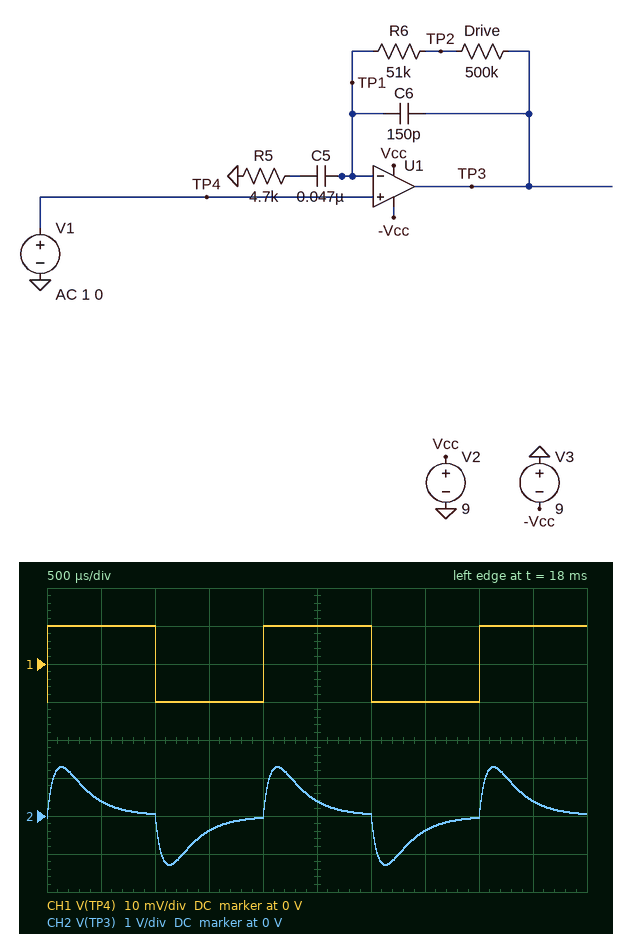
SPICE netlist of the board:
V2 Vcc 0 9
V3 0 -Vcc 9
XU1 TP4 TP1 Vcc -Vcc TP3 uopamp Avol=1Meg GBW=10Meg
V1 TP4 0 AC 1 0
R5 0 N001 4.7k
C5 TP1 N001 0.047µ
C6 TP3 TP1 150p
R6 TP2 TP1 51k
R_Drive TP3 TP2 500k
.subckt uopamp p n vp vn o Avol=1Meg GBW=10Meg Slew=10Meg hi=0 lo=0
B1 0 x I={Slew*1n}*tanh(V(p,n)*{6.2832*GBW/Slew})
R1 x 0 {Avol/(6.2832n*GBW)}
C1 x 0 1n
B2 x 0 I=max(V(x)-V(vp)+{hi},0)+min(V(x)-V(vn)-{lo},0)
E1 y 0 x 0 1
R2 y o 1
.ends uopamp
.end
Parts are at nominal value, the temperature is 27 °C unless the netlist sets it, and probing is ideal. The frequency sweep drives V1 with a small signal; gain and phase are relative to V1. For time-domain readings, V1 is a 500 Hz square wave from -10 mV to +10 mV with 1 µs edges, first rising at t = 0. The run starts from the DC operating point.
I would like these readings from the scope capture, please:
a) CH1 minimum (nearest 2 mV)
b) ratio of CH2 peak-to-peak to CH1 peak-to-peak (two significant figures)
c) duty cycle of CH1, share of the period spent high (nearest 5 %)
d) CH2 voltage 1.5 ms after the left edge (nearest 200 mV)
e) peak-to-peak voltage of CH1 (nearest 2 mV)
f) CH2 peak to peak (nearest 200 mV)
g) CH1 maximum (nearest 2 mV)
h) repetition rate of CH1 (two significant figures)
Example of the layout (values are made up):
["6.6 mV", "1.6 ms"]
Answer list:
["-10 mV", "130", "50 %", "-400 mV", "20 mV", "2.6 V", "10 mV", "500 Hz"]
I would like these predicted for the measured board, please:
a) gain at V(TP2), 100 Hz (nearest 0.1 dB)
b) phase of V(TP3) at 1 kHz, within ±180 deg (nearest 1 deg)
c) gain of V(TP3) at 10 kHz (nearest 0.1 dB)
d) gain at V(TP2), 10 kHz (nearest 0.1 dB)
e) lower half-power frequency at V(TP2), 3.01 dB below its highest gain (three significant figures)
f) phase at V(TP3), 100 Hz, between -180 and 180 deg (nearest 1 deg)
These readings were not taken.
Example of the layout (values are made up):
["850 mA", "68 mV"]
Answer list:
["5.8 dB", "8 deg", "26.8 dB", "7.8 dB", "443 Hz", "76 deg"]
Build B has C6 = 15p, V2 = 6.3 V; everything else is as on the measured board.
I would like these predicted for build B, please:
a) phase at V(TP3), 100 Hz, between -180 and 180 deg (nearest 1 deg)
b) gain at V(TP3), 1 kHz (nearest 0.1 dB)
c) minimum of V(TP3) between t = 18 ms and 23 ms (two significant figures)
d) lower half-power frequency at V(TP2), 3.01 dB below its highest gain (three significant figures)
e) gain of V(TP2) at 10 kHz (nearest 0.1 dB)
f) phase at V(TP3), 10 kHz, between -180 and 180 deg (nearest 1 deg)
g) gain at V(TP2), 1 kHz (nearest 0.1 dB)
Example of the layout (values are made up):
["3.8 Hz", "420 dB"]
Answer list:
["78 deg", "39.7 dB", "-2.0 V", "662 Hz", "20.1 dB", "-28 deg", "19.7 dB"]
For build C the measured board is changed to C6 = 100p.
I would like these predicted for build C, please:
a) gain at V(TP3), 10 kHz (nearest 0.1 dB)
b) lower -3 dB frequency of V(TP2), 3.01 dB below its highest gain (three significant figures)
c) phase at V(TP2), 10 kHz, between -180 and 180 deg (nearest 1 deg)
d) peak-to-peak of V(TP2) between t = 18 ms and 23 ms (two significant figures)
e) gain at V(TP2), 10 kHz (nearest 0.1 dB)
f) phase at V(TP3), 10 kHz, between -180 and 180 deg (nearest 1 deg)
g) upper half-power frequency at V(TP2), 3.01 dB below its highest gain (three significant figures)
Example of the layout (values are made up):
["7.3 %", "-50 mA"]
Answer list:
["30.1 dB", "500 Hz", "-55 deg", "290 mV", "10.6 dB", "-69 deg", "4.03 kHz"]
